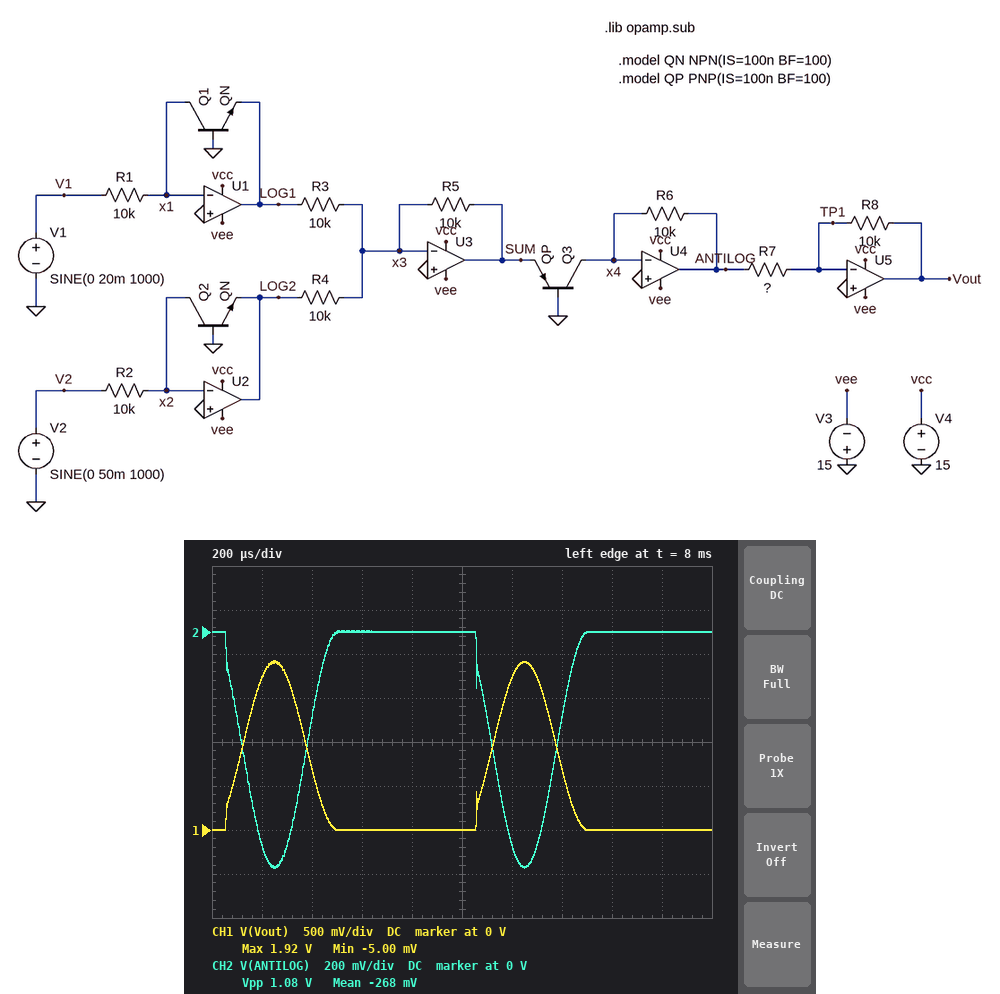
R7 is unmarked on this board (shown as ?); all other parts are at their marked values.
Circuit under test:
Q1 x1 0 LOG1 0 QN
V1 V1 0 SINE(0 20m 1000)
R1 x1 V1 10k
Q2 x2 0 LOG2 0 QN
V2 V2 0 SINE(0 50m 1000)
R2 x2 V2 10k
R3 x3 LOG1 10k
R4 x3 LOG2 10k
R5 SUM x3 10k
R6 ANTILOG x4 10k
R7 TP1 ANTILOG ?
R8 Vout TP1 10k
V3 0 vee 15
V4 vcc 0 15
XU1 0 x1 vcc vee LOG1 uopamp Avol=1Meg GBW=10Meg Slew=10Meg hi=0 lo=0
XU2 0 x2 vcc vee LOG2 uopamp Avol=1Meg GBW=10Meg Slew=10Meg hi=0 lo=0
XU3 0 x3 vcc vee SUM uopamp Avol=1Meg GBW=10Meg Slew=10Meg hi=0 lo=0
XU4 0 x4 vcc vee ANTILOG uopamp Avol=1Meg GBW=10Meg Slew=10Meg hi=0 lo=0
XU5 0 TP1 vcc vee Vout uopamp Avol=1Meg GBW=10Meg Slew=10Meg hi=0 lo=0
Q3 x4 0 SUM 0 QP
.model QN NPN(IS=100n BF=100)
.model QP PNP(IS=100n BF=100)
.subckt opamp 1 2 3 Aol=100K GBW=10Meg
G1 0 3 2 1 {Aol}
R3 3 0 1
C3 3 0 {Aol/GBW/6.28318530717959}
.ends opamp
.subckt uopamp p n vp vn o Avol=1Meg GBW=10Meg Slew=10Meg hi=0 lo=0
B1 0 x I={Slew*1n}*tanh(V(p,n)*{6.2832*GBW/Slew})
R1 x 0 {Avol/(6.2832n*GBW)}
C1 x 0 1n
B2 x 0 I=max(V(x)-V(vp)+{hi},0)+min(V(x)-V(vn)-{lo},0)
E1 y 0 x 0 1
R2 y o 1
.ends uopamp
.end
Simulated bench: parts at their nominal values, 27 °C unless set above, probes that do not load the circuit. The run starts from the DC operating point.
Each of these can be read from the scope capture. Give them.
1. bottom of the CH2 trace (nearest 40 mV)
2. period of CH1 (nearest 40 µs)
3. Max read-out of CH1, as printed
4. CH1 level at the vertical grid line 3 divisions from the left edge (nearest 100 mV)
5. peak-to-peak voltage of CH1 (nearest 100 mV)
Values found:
-1.08 V
1.00 ms
1.92 V
0 V
1.9 V
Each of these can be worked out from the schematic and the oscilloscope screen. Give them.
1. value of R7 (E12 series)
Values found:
5.6 kΩ
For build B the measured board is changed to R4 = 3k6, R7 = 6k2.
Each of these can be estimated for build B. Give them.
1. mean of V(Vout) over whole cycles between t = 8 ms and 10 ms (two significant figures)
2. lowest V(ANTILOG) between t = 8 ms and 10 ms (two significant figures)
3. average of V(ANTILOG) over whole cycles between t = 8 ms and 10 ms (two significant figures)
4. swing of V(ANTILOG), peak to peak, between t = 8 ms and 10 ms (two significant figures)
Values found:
6.2 V
-15 V
-6.1 V
15 V
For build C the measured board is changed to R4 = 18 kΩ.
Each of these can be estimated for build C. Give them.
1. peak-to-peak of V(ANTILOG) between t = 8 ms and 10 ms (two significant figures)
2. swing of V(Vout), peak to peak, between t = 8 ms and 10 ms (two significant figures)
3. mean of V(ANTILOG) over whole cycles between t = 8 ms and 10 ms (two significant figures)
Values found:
190 mV
330 mV
-50 mV
